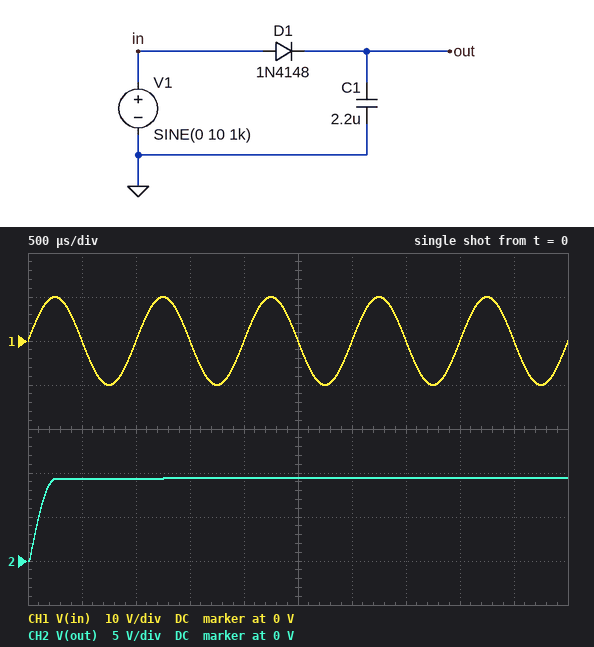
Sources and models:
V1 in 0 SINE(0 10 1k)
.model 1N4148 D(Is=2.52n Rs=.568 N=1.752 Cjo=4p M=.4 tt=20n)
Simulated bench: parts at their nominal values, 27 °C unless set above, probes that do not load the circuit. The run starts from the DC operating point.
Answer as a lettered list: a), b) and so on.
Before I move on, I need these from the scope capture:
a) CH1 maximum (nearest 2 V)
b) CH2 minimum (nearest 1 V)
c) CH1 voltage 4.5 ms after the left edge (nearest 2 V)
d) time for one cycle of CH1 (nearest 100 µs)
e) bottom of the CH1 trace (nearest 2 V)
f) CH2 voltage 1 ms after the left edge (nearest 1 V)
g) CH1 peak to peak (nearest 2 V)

a) 10 V
b) 0 V
c) 0 V
d) 1.0 ms
e) -10 V
f) 9 V
g) 20 V
